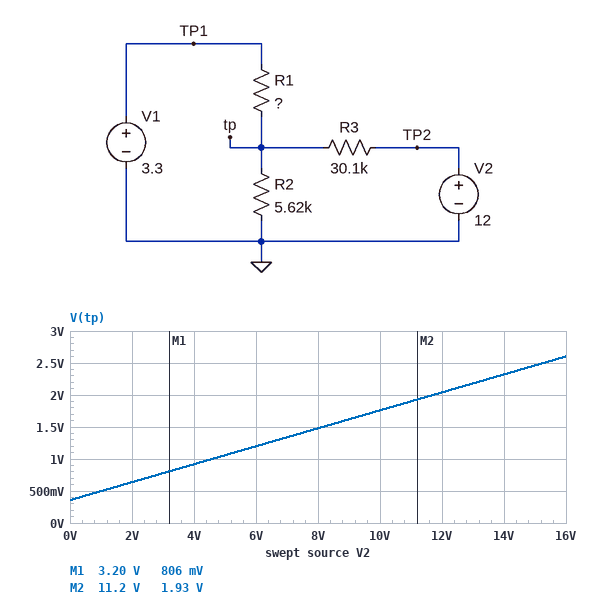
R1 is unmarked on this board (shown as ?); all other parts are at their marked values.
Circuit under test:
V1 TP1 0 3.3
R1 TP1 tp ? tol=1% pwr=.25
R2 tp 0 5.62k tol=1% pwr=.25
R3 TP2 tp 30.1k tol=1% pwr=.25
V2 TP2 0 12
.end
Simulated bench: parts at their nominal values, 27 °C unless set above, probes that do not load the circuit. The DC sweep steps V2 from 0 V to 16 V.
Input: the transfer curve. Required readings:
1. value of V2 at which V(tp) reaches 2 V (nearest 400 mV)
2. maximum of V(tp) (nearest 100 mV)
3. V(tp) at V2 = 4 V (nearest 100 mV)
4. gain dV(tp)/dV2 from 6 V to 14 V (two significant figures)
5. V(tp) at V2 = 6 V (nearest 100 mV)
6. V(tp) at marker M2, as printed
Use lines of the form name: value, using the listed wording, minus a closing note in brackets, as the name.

value of V2 at which V(tp) reaches 2 V: 11.6 V
maximum of V(tp): 2.6 V
V(tp) at V2 = 4 V: 900 mV
gain dV(tp)/dV2 from 6 V to 14 V: 0.14 V/V
V(tp) at V2 = 6 V: 1.2 V
V(tp) at marker M2, as printed: 1.93 V
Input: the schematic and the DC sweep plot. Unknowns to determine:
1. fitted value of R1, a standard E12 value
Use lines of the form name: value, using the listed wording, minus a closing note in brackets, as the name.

fitted value of R1, a standard E12 value: 39 kΩ
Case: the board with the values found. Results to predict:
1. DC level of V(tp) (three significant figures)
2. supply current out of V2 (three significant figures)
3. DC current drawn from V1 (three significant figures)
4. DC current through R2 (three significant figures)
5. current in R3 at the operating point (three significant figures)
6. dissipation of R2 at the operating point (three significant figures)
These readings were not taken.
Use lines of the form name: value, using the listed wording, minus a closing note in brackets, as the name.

DC level of V(tp): 2.04 V
supply current out of V2: 331 µA
DC current drawn from V1: 32.3 µA
DC current through R2: 363 µA
current in R3 at the operating point: 331 µA
dissipation of R2 at the operating point: 741 µW
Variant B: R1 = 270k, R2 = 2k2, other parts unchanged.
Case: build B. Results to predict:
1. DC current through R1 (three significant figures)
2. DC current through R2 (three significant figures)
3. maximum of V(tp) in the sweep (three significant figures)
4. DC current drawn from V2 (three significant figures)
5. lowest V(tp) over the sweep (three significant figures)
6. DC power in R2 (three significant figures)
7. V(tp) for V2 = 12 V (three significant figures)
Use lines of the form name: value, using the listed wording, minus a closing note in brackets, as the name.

DC current through R1: 9.13 µA
DC current through R2: 380 µA
maximum of V(tp) in the sweep: 1.11 V
DC current drawn from V2: 371 µA
lowest V(tp) over the sweep: 24.9 mV
DC power in R2: 318 µW
V(tp) for V2 = 12 V: 836 mV
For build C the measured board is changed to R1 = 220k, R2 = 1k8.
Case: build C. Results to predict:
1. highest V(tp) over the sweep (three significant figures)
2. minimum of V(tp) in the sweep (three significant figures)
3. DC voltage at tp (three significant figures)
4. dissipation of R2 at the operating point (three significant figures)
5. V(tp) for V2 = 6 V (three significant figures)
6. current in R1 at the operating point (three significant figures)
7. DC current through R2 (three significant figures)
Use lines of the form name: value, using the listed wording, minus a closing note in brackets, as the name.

highest V(tp) over the sweep: 921 mV
minimum of V(tp) in the sweep: 25.3 mV
DC voltage at tp: 697 mV
dissipation of R2 at the operating point: 270 µW
V(tp) for V2 = 6 V: 361 mV
current in R1 at the operating point: 11.8 µA
DC current through R2: 387 µA
